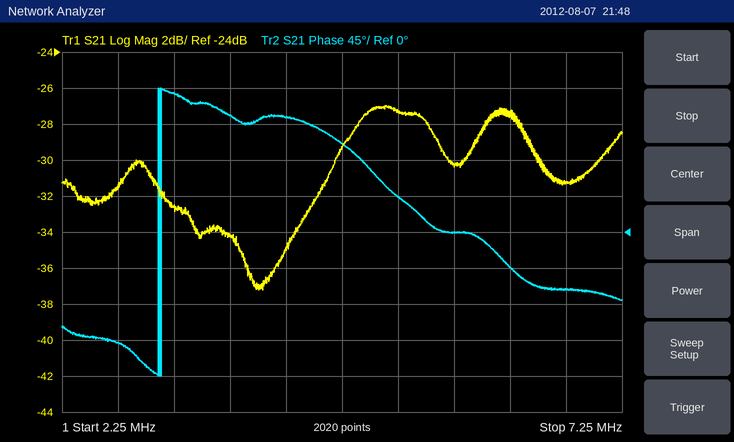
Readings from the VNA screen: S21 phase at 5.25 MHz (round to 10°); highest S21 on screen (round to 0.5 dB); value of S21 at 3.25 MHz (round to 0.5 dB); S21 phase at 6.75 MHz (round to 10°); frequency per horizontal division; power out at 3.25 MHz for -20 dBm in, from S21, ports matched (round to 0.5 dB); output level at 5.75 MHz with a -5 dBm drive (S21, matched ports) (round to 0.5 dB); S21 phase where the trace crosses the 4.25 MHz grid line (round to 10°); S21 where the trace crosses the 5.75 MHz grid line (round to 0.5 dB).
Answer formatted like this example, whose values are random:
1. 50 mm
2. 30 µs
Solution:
1. 40°
2. -27.0 dB
3. -32.5 dB
4. -70°
5. 500 kHz
6. -52.5 dBm
7. -35.5 dBm
8. 140°
9. -30.5 dB
